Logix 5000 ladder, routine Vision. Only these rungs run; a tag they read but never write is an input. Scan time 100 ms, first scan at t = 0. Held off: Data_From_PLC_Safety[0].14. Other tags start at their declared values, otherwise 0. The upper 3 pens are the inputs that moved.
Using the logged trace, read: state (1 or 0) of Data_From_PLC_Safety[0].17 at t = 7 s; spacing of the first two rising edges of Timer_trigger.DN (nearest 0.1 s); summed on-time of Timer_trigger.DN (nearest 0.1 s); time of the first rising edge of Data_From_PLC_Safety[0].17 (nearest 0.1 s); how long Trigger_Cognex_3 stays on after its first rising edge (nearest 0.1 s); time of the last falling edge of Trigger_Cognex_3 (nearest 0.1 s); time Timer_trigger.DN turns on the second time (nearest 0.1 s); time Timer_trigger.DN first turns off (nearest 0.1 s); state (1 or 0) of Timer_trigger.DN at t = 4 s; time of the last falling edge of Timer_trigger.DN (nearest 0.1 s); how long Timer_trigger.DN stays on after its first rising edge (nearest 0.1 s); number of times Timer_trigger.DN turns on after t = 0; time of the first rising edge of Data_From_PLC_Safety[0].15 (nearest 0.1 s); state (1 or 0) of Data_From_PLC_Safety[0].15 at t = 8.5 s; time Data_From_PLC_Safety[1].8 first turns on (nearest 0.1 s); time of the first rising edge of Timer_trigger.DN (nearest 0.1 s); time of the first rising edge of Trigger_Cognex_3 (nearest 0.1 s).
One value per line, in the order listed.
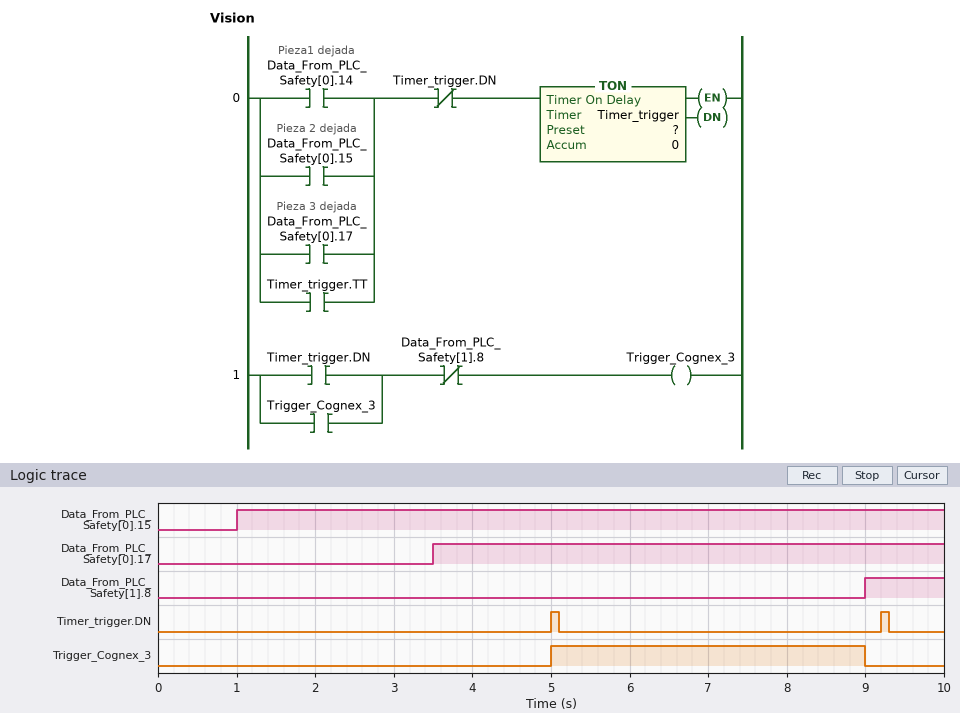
1
4.2 s
0.2 s
3.5 s
4.0 s
9.0 s
9.2 s
5.1 s
0
9.3 s
0.1 s
2
1.0 s
1
9.0 s
5.0 s
5.0 s
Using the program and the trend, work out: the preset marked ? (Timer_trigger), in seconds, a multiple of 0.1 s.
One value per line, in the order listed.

4.0 s
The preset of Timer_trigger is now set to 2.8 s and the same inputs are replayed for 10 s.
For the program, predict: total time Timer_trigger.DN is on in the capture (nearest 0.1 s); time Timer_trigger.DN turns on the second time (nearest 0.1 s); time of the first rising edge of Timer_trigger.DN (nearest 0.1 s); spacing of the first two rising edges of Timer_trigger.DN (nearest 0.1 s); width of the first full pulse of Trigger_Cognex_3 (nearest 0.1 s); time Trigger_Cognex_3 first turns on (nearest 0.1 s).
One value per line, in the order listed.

0.3 s
6.8 s
3.8 s
3.0 s
5.2 s
3.8 s
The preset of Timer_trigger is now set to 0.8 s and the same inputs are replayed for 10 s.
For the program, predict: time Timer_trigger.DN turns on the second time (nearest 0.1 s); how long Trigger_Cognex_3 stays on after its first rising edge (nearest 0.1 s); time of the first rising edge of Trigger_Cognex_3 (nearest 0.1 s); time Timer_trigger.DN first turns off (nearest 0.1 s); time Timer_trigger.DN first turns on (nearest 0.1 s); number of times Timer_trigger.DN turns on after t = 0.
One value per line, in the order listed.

2.8 s
7.2 s
1.8 s
1.9 s
1.8 s
9
